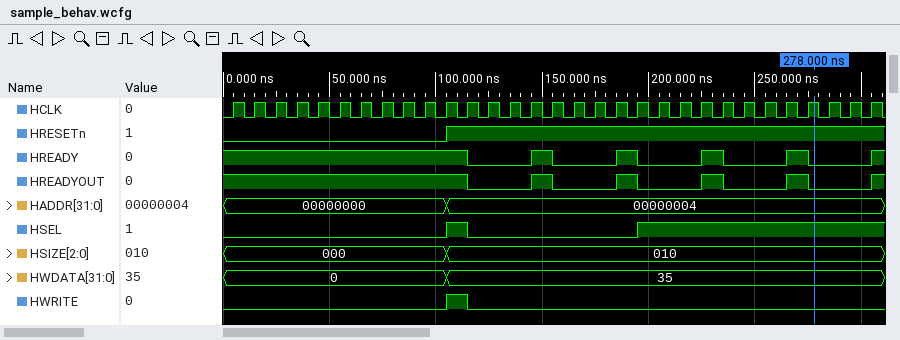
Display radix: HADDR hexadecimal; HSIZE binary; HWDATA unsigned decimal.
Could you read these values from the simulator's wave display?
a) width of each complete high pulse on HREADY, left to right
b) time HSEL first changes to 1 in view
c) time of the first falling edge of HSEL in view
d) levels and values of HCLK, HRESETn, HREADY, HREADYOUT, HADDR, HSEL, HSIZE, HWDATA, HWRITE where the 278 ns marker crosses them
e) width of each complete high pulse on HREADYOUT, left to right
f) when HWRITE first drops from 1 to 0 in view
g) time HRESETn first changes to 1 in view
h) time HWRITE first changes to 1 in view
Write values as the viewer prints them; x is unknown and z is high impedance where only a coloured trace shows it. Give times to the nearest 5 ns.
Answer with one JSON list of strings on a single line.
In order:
["10 ns, 10 ns, 10 ns, 10 ns", "105 ns", "115 ns", "HCLK=1, HRESETn=1, HREADY=0, HREADYOUT=0, HADDR=00000004, HSEL=1, HSIZE=010, HWDATA=35, HWRITE=0", "10 ns, 10 ns, 10 ns, 10 ns", "115 ns", "105 ns", "105 ns"]
